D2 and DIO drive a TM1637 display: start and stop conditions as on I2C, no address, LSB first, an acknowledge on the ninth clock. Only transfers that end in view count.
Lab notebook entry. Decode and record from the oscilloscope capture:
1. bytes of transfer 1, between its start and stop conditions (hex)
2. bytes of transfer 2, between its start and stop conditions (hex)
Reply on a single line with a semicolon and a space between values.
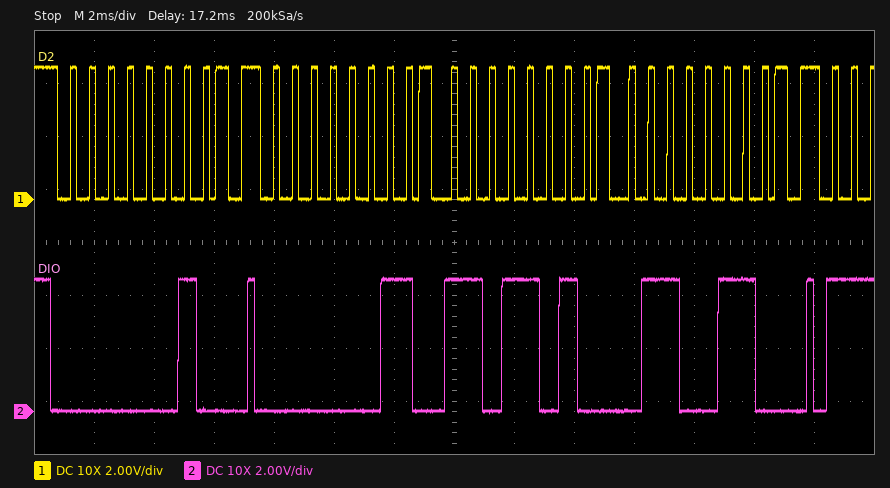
40; C0 5B 66
